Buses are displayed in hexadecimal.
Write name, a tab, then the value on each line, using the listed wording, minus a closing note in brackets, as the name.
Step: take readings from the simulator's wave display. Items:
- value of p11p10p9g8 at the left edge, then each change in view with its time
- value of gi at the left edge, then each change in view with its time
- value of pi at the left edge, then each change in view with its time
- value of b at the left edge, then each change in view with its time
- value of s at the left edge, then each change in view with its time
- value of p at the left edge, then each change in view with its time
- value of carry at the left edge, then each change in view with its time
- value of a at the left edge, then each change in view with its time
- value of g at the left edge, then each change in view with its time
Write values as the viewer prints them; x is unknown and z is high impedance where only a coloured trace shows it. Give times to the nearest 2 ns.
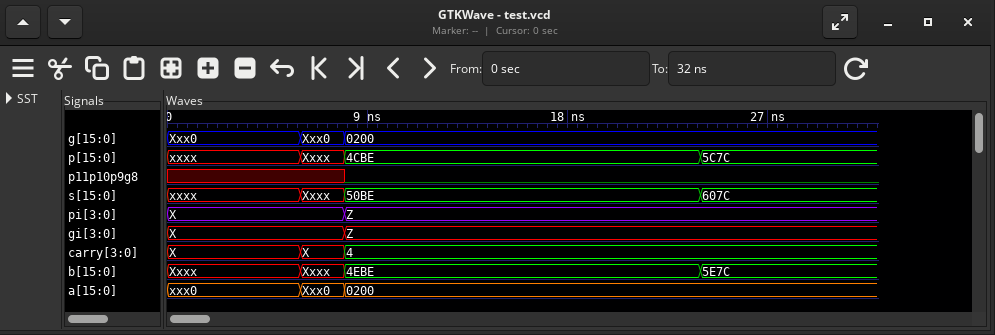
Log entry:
value of p11p10p9g8 at the left edge, then each change in view with its time	x, 0 at 8 ns
value of gi at the left edge, then each change in view with its time	X, Z at 8 ns
value of pi at the left edge, then each change in view with its time	X, Z at 8 ns
value of b at the left edge, then each change in view with its time	Xxxx, Xxxx at 6 ns, 4EBE at 8 ns, 5E7C at 24 ns
value of s at the left edge, then each change in view with its time	xxxx, Xxxx at 6 ns, 50BE at 8 ns, 607C at 24 ns
value of p at the left edge, then each change in view with its time	xxxx, Xxxx at 6 ns, 4CBE at 8 ns, 5C7C at 24 ns
value of carry at the left edge, then each change in view with its time	X, X at 6 ns, 4 at 8 ns
value of a at the left edge, then each change in view with its time	xxx0, Xxx0 at 6 ns, 0200 at 8 ns
value of g at the left edge, then each change in view with its time	Xxx0, Xxx0 at 6 ns, 0200 at 8 ns
